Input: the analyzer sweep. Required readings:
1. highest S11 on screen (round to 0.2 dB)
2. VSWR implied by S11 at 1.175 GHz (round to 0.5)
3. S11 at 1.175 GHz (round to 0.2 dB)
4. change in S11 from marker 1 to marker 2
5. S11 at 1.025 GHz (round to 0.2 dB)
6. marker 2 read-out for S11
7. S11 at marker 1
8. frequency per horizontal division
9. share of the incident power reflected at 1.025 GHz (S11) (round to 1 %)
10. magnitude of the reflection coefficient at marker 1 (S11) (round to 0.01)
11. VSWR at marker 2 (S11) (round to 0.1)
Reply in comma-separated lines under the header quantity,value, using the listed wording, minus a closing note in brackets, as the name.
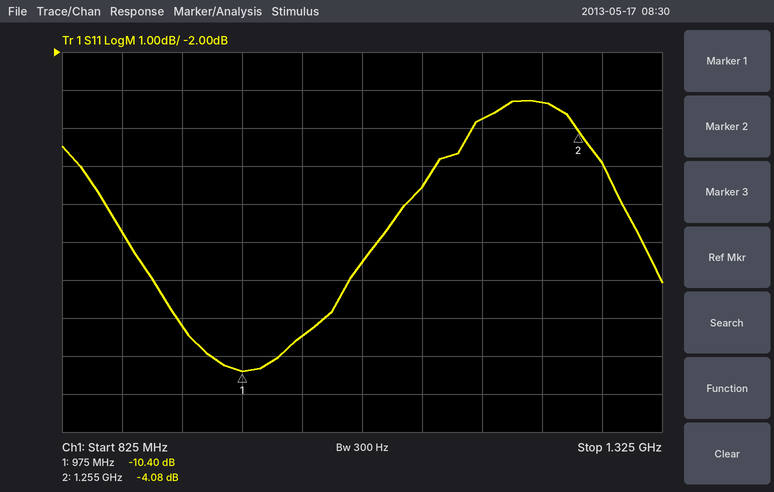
quantity,value
highest S11 on screen,-3.2 dB
VSWR implied by S11 at 1.175 GHz,4.5
S11 at 1.175 GHz,-3.8 dB
change in S11 from marker 1 to marker 2,6.32 dB
S11 at 1.025 GHz,-9.4 dB
marker 2 read-out for S11,-4.08 dB
S11 at marker 1,-10.40 dB
frequency per horizontal division,50 MHz
share of the incident power reflected at 1.025 GHz (S11),11 %
magnitude of the reflection coefficient at marker 1 (S11),0.30
VSWR at marker 2 (S11),4.3
